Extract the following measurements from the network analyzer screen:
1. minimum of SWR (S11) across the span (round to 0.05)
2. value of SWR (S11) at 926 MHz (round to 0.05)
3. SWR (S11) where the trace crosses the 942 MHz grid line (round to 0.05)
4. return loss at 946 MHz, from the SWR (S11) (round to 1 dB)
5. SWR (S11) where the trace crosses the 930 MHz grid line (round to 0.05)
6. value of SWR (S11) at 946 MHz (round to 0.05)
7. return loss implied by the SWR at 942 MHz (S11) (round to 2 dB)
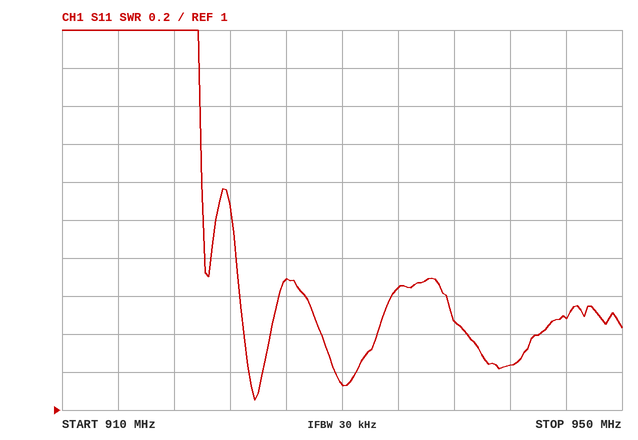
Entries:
1.05
1.70
1.25
14 dB
1.15
1.50
20 dB
